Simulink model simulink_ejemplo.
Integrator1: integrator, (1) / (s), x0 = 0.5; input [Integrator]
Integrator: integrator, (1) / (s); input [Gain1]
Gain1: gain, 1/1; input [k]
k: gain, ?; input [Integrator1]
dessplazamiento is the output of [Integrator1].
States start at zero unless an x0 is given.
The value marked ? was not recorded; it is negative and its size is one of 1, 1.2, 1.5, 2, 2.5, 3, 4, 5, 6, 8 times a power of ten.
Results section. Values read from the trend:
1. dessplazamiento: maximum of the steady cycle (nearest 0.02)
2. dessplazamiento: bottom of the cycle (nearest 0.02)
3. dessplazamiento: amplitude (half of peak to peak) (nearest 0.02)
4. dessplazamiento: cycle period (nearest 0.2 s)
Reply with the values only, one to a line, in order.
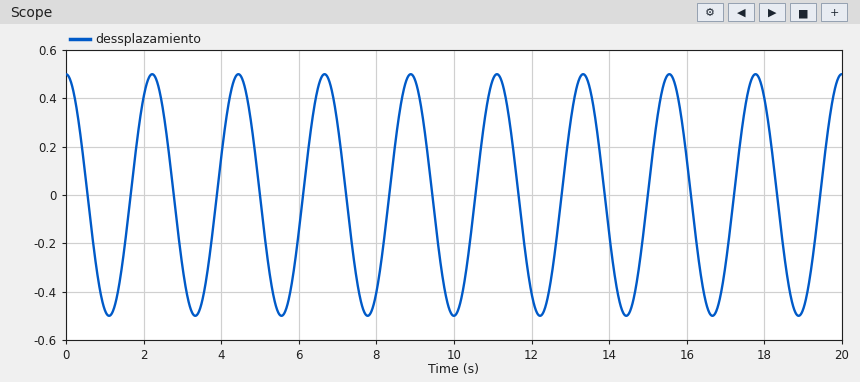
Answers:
0.50
-0.50
0.50
2.2 s
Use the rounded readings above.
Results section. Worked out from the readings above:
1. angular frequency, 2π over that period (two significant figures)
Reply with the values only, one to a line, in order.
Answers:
2.9 rad/s
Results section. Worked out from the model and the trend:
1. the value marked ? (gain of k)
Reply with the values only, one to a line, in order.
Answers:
-8
